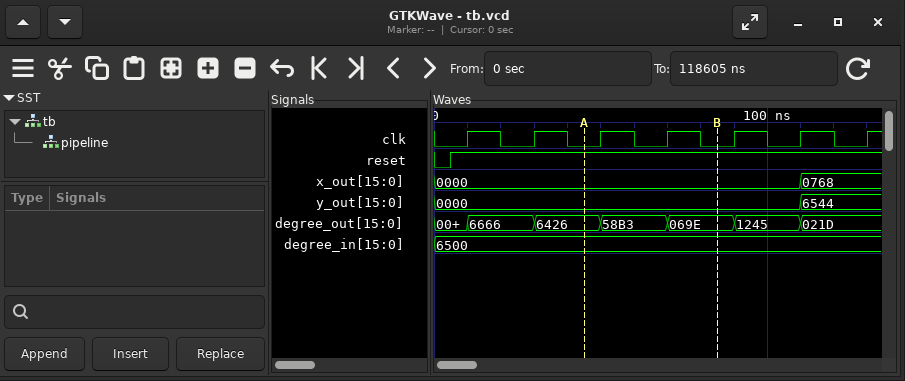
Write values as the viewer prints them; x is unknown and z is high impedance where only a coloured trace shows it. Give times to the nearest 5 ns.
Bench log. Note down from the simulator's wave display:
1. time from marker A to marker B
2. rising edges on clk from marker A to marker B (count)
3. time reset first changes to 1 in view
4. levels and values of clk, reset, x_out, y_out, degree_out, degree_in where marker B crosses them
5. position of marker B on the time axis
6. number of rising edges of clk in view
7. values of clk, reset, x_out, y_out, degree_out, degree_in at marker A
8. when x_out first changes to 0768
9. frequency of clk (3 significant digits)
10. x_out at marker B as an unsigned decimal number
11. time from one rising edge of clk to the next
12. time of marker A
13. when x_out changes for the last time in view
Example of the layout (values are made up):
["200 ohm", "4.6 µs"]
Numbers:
["40 ns", "2", "5 ns", "clk=0, reset=1, x_out=0000, y_out=0000, degree_out=069E, degree_in=6500", "85 ns", "7", "clk=0, reset=1, x_out=0000, y_out=0000, degree_out=6426, degree_in=6500", "110 ns", "50.0 MHz", "0", "20 ns", "45 ns", "110 ns"]
